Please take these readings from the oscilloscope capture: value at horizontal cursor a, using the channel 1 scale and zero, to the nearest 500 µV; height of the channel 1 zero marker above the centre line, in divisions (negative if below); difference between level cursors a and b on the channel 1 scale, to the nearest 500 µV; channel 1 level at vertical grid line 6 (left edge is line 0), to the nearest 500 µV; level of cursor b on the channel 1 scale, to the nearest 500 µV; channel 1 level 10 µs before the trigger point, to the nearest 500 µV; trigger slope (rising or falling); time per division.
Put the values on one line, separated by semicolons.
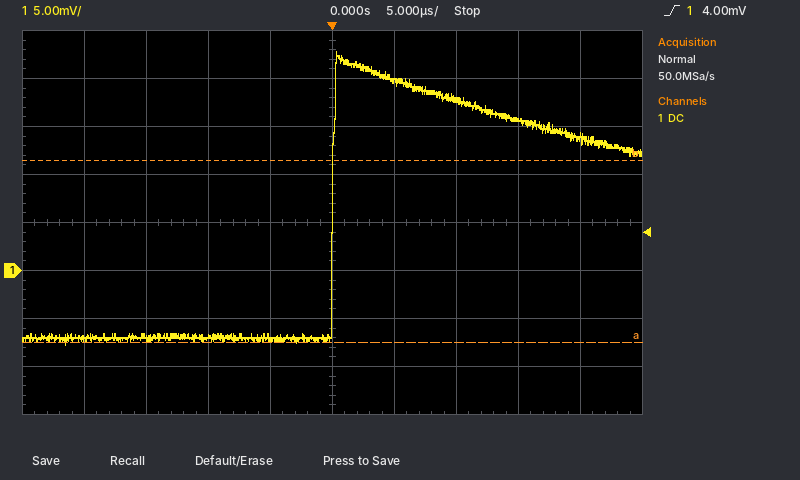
-7.5 mV; -1.0 div; 19.0 mV; 19.5 mV; 11.5 mV; -7.0 mV; rising; 5 µs
